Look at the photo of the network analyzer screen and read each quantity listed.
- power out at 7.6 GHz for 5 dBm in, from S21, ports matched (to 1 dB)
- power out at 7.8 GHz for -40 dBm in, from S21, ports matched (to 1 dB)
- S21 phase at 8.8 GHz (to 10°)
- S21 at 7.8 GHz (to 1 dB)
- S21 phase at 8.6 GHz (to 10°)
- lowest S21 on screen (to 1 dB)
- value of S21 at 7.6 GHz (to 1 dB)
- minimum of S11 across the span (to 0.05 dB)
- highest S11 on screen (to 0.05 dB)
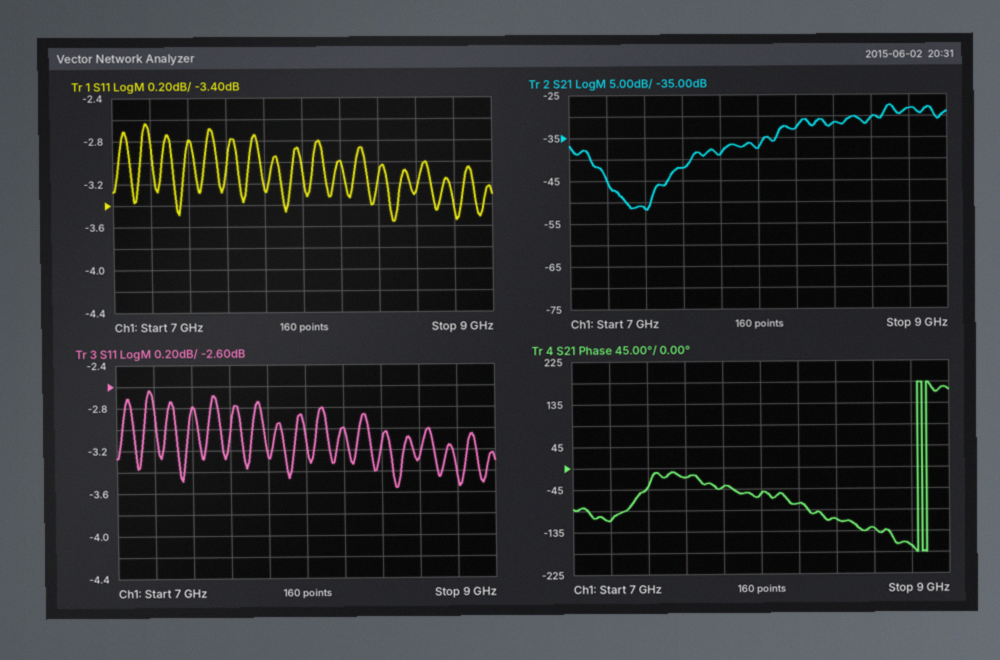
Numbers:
-37 dBm
-79 dBm
-170°
-39 dB
-130°
-52 dB
-42 dB
-3.55 dB
-2.65 dB
